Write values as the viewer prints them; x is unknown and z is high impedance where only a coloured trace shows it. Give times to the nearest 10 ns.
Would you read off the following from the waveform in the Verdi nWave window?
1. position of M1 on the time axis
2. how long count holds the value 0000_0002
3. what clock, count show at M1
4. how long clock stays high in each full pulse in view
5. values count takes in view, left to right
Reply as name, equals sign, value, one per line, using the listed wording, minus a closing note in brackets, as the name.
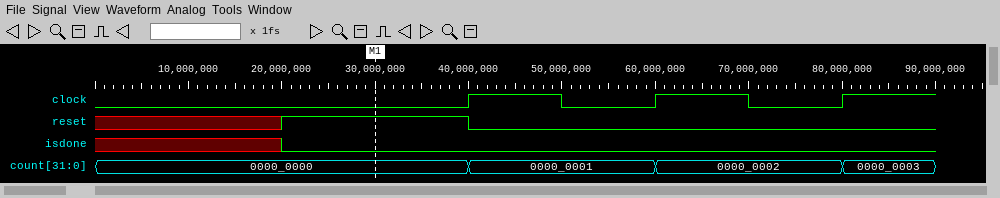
position of M1 on the time axis = 30 ns
how long count holds the value 0000_0002 = 20 ns
what clock, count show at M1 = clock=0, count=0000_0000
how long clock stays high in each full pulse in view = 10 ns, 10 ns
values count takes in view, left to right = 0000_0000, 0000_0001, 0000_0002, 0000_0003
